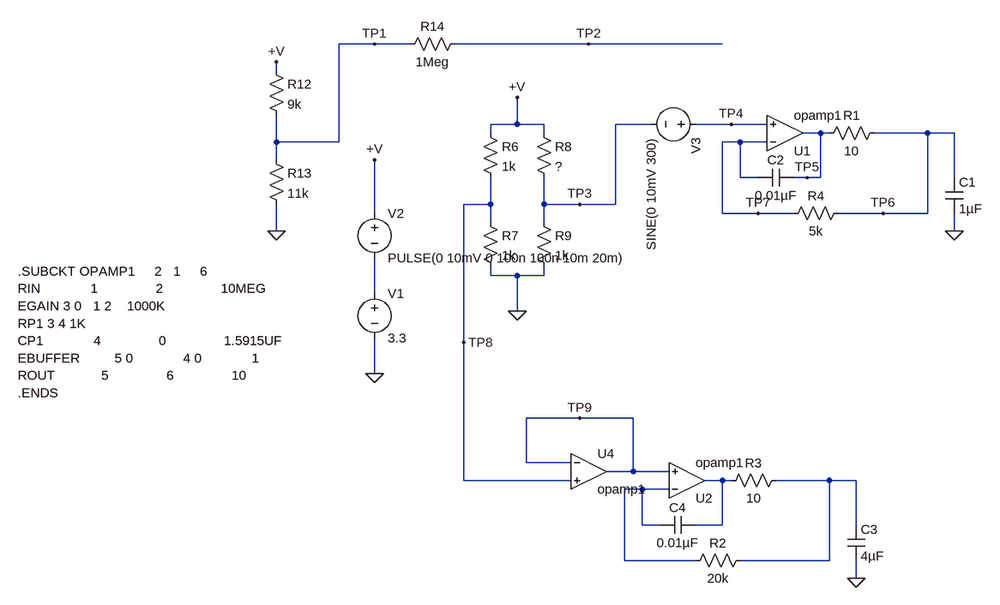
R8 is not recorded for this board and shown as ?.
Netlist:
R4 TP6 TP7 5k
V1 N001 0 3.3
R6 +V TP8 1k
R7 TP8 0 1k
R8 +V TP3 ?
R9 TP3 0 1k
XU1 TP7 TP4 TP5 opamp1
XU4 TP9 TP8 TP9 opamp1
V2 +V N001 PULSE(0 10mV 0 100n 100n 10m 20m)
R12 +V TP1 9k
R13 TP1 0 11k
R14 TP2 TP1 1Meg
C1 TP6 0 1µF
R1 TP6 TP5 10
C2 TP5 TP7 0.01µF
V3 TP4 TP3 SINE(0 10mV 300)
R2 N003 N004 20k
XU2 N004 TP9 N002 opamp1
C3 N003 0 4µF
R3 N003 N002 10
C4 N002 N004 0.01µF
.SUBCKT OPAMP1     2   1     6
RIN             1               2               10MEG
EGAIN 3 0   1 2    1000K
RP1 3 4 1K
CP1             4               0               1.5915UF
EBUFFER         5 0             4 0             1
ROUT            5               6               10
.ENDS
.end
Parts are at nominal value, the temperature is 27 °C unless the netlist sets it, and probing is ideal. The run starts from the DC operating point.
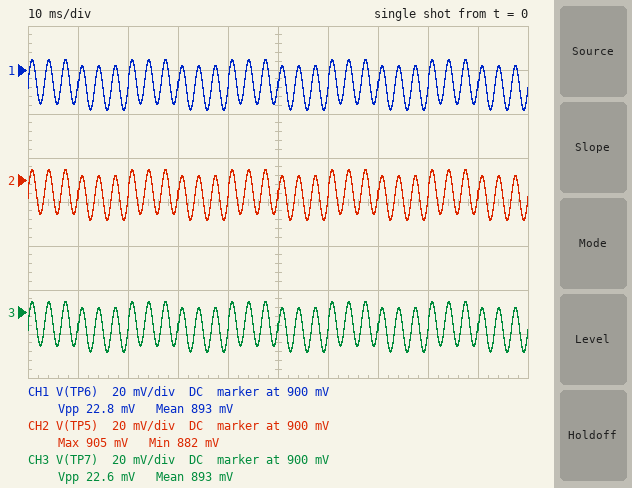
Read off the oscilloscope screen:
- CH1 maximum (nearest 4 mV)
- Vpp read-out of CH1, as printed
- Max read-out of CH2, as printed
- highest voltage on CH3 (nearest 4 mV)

904 mV
22.8 mV
905 mV
904 mV
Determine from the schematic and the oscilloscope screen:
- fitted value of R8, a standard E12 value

2.7 kΩ
